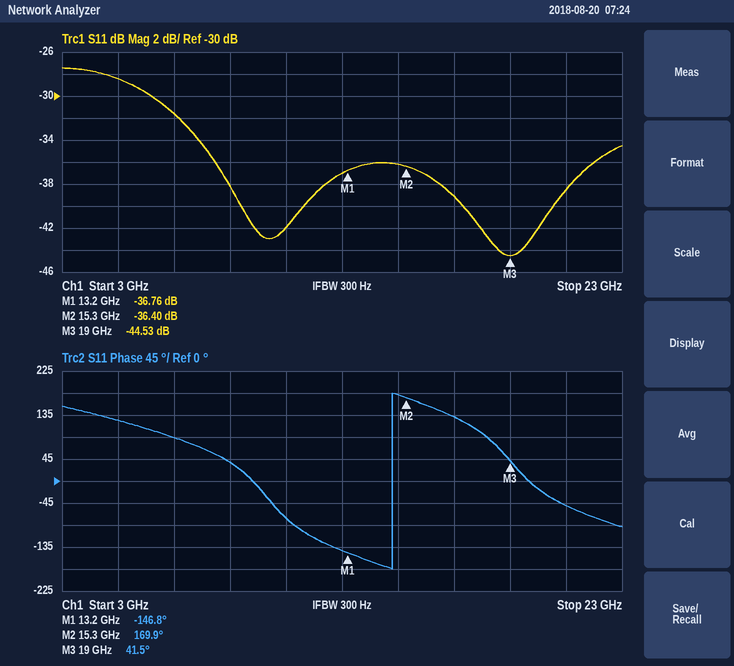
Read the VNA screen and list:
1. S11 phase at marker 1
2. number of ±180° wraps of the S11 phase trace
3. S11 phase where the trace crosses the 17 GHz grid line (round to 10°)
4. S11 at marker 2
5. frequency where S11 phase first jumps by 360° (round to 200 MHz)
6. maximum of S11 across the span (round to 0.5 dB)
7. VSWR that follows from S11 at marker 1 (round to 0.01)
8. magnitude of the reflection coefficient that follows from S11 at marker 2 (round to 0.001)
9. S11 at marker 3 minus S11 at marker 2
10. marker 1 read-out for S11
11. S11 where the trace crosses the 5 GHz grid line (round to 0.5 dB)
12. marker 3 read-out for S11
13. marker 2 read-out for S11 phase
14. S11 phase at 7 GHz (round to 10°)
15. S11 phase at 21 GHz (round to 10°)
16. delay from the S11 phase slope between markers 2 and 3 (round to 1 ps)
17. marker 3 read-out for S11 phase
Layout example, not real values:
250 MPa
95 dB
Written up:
-146.8°
1
130°
-36.40 dB
14.8 GHz
-27.5 dB
1.03
0.015
-8.13 dB
-36.76 dB
-28.5 dB
-44.53 dB
169.9°
90°
-50°
96 ps
41.5°
